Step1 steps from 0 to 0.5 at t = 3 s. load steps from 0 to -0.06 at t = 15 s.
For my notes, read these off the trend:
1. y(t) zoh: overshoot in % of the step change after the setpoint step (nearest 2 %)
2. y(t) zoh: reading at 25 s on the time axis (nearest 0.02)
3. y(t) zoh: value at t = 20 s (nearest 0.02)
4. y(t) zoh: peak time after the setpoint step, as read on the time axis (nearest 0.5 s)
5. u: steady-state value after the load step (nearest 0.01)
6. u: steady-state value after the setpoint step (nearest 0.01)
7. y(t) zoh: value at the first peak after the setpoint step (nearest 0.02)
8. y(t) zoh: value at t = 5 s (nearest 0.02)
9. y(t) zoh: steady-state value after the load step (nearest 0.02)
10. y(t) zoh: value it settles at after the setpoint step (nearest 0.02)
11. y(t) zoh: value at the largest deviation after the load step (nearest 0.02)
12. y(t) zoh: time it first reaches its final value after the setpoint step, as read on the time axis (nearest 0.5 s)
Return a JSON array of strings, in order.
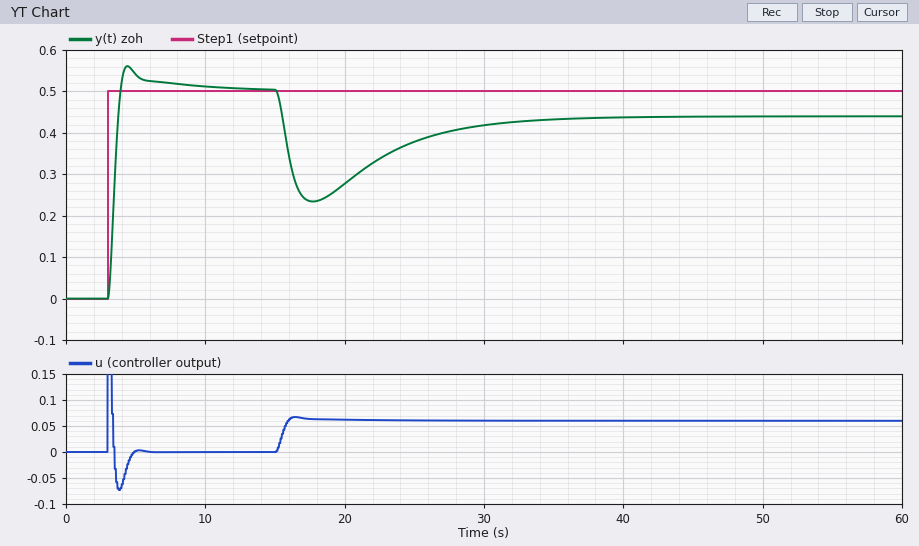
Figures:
["12 %", "0.38", "0.28", "4.5 s", "0.06", "0.00", "0.56", "0.54", "0.44", "0.50", "0.24", "4.0 s"]
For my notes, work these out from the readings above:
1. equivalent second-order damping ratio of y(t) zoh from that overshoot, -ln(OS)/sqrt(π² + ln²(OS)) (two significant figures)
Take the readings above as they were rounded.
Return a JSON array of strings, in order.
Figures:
["0.56"]
